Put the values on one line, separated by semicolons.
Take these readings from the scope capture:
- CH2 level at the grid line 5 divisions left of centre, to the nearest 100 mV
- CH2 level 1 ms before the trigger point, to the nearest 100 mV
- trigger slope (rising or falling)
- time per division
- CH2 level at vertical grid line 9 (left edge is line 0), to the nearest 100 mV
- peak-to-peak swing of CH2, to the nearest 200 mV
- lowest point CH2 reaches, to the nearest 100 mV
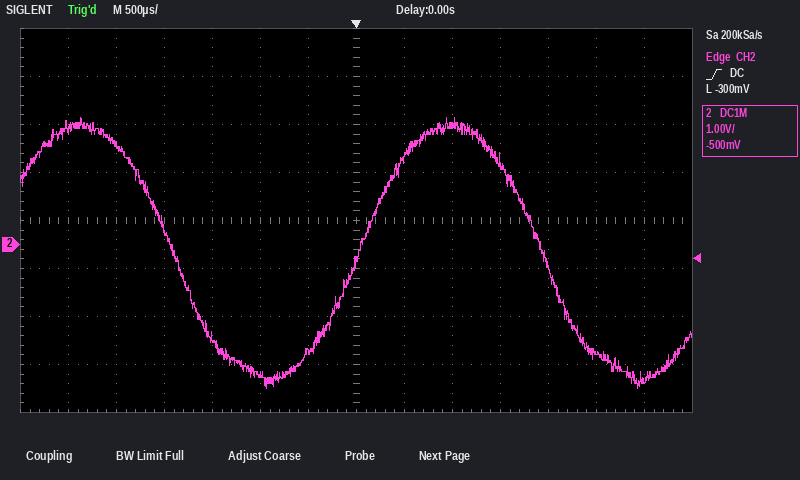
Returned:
2.1 V; -2.7 V; rising; 500 µs; 2.5 V; 5.6 V; -3.0 V
